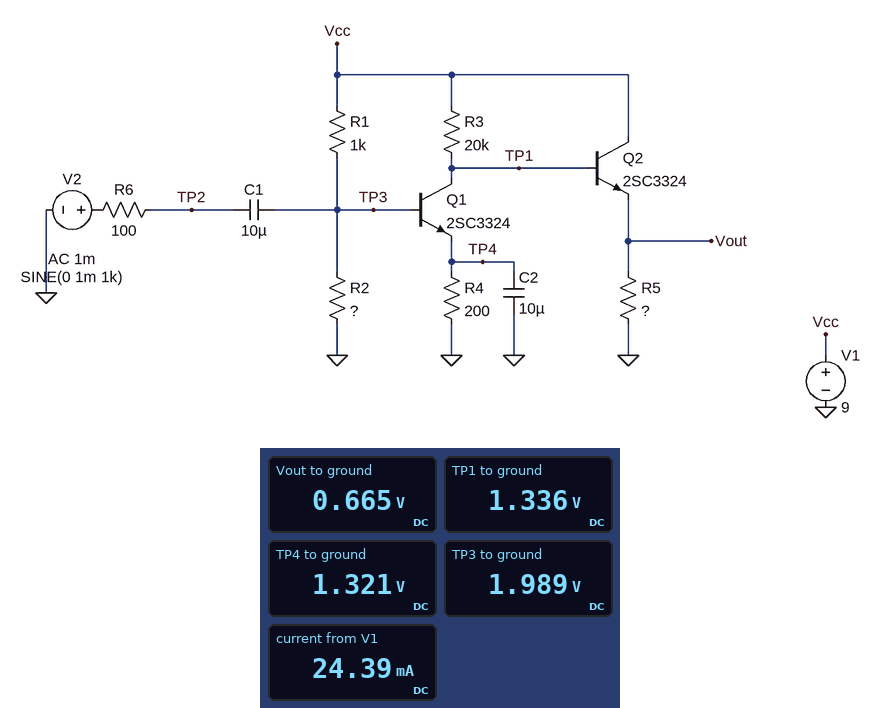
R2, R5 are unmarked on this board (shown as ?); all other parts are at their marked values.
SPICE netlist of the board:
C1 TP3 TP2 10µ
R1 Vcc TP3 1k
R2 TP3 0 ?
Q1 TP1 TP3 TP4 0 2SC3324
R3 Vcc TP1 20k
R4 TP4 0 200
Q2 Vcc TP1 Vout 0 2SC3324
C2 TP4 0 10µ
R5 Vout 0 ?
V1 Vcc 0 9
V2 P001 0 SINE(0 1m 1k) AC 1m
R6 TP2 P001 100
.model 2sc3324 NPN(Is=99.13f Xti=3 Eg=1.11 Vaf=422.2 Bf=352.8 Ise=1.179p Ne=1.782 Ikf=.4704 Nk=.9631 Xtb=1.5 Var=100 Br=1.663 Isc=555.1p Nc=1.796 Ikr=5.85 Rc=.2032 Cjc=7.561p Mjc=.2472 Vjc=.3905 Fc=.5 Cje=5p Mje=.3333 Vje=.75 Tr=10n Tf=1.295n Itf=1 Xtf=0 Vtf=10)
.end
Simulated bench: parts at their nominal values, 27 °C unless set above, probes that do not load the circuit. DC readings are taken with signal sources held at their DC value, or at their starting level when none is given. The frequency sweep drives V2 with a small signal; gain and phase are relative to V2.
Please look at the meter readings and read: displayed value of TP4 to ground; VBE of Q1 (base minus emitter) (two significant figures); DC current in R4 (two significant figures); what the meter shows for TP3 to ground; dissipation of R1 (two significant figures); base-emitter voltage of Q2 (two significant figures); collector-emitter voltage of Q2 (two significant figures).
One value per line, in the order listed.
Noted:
1.321 V
670 mV
6.6 mA
1.989 V
49 mW
670 mV
8.3 V
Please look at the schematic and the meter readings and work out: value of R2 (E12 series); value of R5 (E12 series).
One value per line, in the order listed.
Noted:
2.7 kΩ
39 Ω
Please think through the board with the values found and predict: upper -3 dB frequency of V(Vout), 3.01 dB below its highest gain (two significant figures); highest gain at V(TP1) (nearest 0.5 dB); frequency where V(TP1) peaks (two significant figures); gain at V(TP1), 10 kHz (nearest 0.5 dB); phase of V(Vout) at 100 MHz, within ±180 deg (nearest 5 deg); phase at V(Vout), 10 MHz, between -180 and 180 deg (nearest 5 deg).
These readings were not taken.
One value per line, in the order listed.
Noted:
440 Hz
-8.5 dB
130 Hz
-36.5 dB
-30 deg
40 deg
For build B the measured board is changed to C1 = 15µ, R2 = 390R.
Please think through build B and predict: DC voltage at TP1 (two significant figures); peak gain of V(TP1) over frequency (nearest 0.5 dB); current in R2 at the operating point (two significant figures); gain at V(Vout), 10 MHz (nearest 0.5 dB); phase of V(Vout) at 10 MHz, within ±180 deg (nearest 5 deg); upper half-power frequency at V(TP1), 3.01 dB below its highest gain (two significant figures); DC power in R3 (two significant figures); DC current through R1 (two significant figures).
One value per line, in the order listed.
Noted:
840 mV
-8.5 dB
3.8 mA
-36.0 dB
50 deg
410 Hz
3.3 mW
7.5 mA
